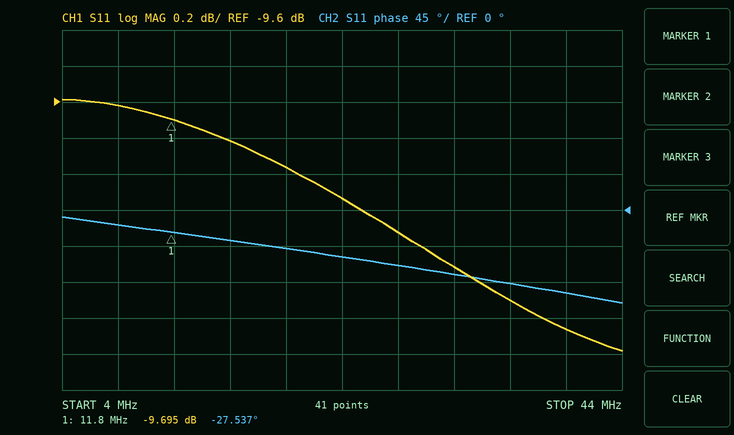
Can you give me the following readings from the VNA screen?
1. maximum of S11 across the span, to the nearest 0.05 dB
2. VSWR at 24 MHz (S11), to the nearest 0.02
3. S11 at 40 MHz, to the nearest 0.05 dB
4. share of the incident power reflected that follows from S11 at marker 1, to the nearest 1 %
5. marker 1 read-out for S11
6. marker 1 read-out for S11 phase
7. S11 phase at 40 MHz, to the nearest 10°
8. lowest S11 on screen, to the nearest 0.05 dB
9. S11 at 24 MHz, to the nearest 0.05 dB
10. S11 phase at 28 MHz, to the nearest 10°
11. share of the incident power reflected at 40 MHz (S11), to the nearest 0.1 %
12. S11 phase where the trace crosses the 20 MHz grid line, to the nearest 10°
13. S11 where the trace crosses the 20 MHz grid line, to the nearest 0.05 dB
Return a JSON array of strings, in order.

["-9.60 dB", "1.90", "-10.85 dB", "11 %", "-9.695 dB", "-27.537°", "-100°", "-11.00 dB", "-10.15 dB", "-70°", "8.2 %", "-50°", "-9.95 dB"]
